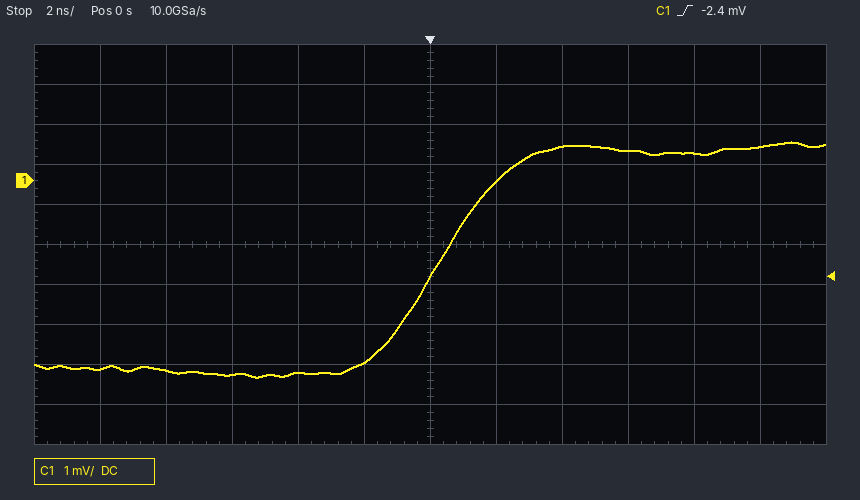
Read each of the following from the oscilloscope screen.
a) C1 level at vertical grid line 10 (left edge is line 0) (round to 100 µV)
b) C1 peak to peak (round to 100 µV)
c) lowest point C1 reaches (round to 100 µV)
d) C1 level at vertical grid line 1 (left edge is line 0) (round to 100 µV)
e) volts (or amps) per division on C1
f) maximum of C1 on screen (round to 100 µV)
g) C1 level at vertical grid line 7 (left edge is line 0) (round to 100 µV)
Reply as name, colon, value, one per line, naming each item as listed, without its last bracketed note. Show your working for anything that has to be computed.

C1 level at vertical grid line 10 (left edge is line 0): 700 µV
C1 peak to peak: 1.0 mV − (-4.9 mV) = 5.9 mV
lowest point C1 reaches: -4.9 mV
C1 level at vertical grid line 1 (left edge is line 0): -4.7 mV
volts (or amps) per division on C1: 1 mV
maximum of C1 on screen: 1.0 mV
C1 level at vertical grid line 7 (left edge is line 0): 0.0 mV
